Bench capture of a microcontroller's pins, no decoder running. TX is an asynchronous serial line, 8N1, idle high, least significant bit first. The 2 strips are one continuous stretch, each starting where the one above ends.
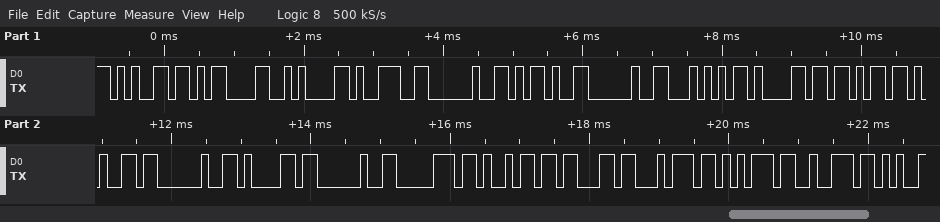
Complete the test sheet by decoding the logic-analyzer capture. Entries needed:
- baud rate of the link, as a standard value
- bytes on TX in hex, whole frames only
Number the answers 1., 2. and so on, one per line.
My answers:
1. 9600 baud
2. 65 0D 0A 39 20 2D 20 54 61 6B 65 20 61 20 70 69 63 74 75 72
